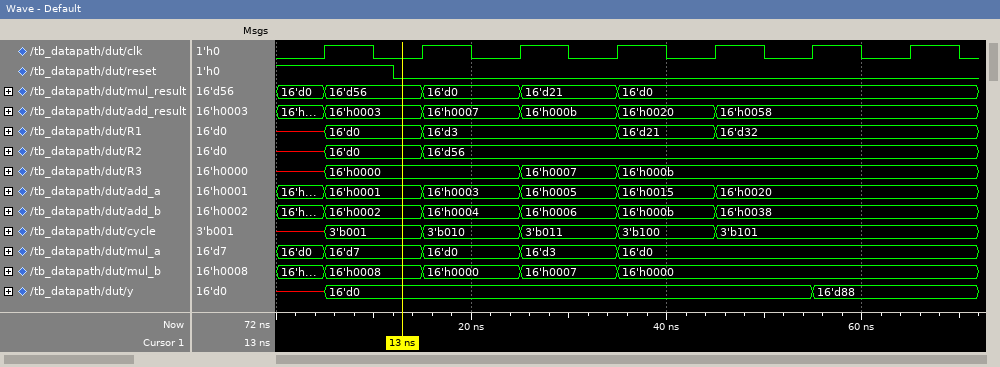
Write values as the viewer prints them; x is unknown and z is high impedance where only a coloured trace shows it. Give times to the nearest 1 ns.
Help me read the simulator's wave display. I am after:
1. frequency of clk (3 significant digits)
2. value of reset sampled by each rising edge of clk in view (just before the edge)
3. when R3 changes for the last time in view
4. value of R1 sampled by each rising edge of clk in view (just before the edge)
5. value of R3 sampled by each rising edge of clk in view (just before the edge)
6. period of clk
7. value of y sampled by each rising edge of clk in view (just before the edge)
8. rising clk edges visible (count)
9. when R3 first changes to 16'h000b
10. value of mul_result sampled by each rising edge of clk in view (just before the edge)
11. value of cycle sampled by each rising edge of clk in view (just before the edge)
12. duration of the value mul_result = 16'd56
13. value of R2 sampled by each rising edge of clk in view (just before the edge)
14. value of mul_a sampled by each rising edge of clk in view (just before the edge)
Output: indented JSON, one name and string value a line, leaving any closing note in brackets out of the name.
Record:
{
  "frequency of clk": "100 MHz",
  "value of reset sampled by each rising edge of clk in view": "1 0 0 0 0 0 0",
  "when R3 changes for the last time in view": "35 ns",
  "value of R1 sampled by each rising edge of clk in view": "x, 16'd0, 16'd3, 16'd3, 16'd21, 16'd32, 16'd32",
  "value of R3 sampled by each rising edge of clk in view": "x, 16'h0000, 16'h0000, 16'h0007, 16'h000b, 16'h000b, 16'h000b",
  "period of clk": "10 ns",
  "value of y sampled by each rising edge of clk in view": "x, 16'd0, 16'd0, 16'd0, 16'd0, 16'd0, 16'd88",
  "rising clk edges visible": "7",
  "when R3 first changes to 16'h000b": "35 ns",
  "value of mul_result sampled by each rising edge of clk in view": "16'd0, 16'd56, 16'd0, 16'd21, 16'd0, 16'd0, 16'd0",
  "value of cycle sampled by each rising edge of clk in view": "x, 3'b001, 3'b010, 3'b011, 3'b100, 3'b101, 3'b101",
  "duration of the value mul_result = 16'd56": "10 ns",
  "value of R2 sampled by each rising edge of clk in view": "x, 16'd0, 16'd56, 16'd56, 16'd56, 16'd56, 16'd56",
  "value of mul_a sampled by each rising edge of clk in view": "16'd0, 16'd7, 16'd0, 16'd3, 16'd0, 16'd0, 16'd0"
}
